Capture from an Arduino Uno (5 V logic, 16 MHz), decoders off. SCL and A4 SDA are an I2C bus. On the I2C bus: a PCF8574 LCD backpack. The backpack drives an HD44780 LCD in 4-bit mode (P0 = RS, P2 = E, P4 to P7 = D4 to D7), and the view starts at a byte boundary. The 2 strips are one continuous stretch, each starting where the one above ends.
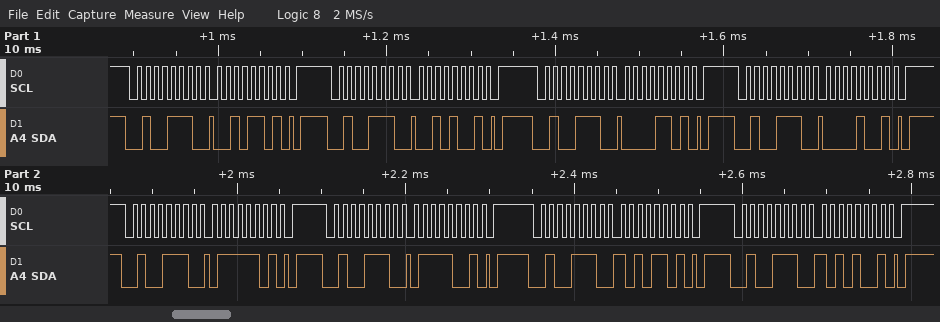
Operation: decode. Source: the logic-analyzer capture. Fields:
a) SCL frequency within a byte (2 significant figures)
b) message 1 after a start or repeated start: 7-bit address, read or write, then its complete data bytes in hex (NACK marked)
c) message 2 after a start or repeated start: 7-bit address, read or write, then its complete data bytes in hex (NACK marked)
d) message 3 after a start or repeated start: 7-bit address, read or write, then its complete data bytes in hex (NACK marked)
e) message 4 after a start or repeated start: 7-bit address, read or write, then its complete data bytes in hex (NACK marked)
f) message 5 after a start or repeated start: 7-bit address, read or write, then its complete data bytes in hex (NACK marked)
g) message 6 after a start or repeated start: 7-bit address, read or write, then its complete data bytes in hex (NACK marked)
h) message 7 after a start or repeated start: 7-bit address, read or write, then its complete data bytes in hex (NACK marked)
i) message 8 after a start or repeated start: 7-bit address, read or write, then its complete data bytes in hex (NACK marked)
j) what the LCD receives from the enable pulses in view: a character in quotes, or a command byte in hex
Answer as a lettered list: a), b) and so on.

a) 100 kHz
b) 0x27 write: 2D
c) 0x27 write: 29
d) 0x27 write: 0D
e) 0x27 write: 09
f) 0x27 write: 7D
g) 0x27 write: 79
h) 0x27 write: AD
i) 0x27 write: A9
j) ' ' 'z'
